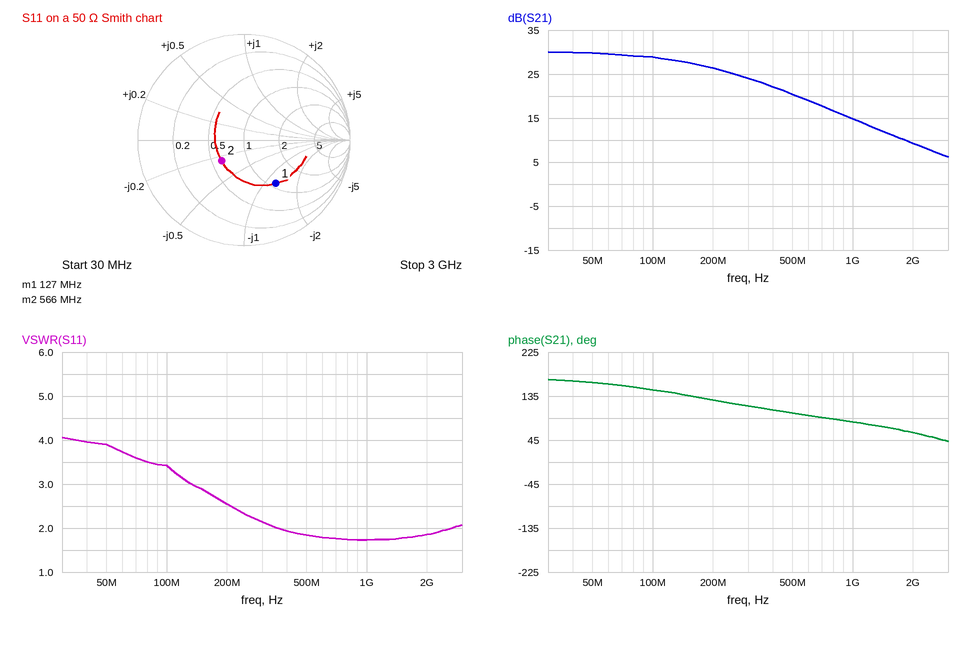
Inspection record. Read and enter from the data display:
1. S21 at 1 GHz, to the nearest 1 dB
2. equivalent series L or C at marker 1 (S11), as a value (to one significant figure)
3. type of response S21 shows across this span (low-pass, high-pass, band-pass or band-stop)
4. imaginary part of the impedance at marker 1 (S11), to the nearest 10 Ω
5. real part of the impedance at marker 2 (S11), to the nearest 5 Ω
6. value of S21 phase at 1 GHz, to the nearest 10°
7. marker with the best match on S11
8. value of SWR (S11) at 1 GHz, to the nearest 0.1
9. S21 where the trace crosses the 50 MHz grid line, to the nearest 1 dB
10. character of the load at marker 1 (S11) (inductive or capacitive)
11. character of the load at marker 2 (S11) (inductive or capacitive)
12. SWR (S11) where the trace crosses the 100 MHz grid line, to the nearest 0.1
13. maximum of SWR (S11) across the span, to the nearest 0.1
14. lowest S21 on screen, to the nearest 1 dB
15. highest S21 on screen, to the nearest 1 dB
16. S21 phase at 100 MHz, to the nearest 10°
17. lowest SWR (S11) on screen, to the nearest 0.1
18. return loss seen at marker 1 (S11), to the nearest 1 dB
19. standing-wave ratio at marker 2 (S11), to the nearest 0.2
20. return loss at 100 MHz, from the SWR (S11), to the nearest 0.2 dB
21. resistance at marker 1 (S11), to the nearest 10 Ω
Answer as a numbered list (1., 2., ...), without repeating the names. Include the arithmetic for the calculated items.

1. 15 dB
2. C = 1/(2π × 127 MHz × 60 Ω) ≈ 20.9 pF, so 20 pF to one significant figure
3. low-pass
4. -60 Ω
5. 30 Ω
6. 80°
7. marker 2
8. 1.7
9. 30 dB
10. capacitive
11. capacitive
12. 3.4
13. 4.1
14. 6 dB
15. 30 dB
16. 150°
17. 1.7
18. 6 dB
19. 1.8
20. −20 log10((3.4 − 1)/(3.4 + 1)) ≈ 5.26 dB, so 5.2 dB to the nearest 0.2 dB
21. 60 Ω
